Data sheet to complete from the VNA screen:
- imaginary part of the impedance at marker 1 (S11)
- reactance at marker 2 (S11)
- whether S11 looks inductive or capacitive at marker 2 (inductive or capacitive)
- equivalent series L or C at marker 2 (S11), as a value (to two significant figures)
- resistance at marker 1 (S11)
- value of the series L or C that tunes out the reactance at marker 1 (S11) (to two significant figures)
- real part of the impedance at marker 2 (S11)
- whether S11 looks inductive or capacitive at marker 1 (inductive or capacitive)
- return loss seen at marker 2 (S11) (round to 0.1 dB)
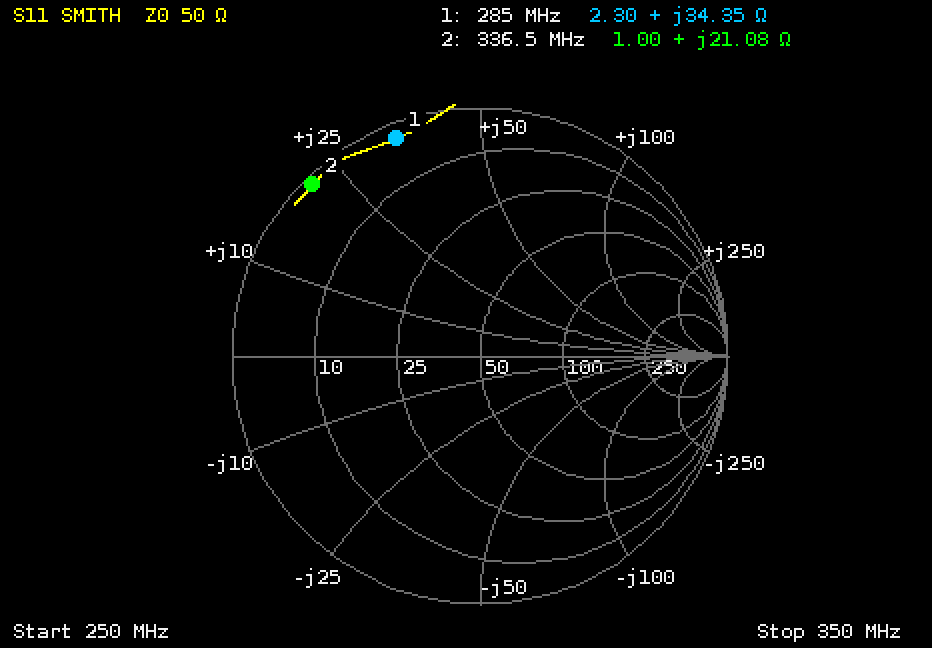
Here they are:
+34.35 Ω
+21.08 Ω
inductive
10.0 nH
2.30 Ω
16 pF
1.00 Ω
inductive
0.3 dB
